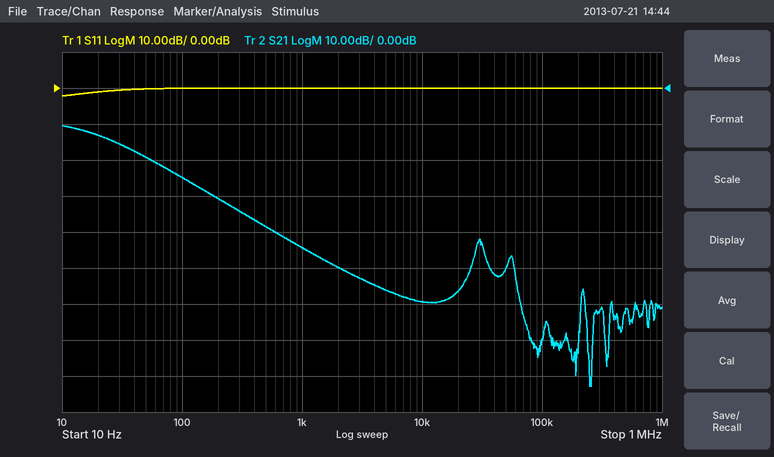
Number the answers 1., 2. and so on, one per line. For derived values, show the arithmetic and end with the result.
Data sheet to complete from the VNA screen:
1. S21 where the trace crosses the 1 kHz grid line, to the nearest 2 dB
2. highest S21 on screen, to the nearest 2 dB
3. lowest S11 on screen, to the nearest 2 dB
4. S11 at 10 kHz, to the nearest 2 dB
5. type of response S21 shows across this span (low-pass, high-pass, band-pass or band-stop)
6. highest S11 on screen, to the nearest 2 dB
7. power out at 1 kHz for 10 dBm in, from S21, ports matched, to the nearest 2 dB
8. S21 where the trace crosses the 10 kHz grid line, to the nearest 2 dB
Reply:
1. -44 dB
2. -10 dB
3. -2 dB
4. 0 dB
5. low-pass
6. 0 dB
7. 10 dBm + (-44 dB) = -34 dBm
8. -60 dB
